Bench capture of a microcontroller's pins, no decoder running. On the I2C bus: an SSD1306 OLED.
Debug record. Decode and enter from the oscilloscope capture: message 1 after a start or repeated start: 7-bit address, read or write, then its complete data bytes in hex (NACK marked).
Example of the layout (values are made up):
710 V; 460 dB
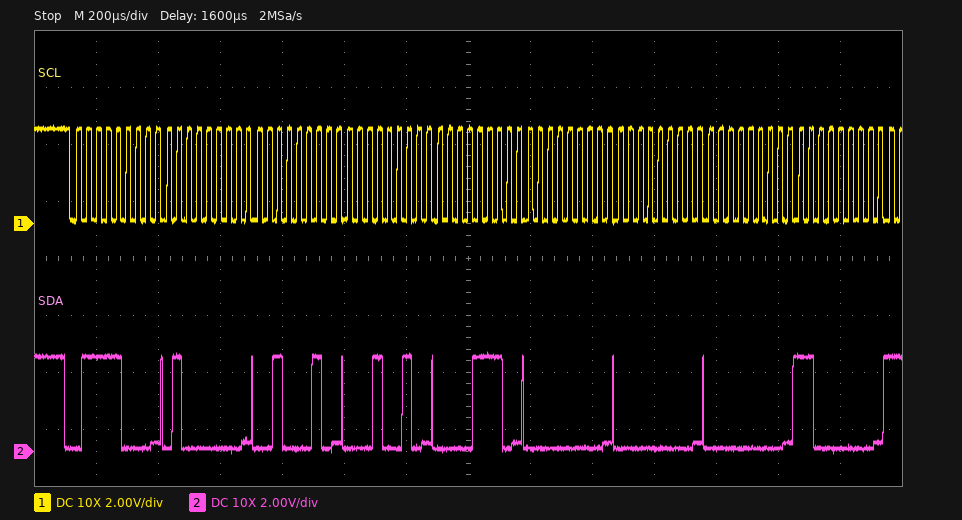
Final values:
0x3C write: 40 22 12 0E 00 00 00 C0
